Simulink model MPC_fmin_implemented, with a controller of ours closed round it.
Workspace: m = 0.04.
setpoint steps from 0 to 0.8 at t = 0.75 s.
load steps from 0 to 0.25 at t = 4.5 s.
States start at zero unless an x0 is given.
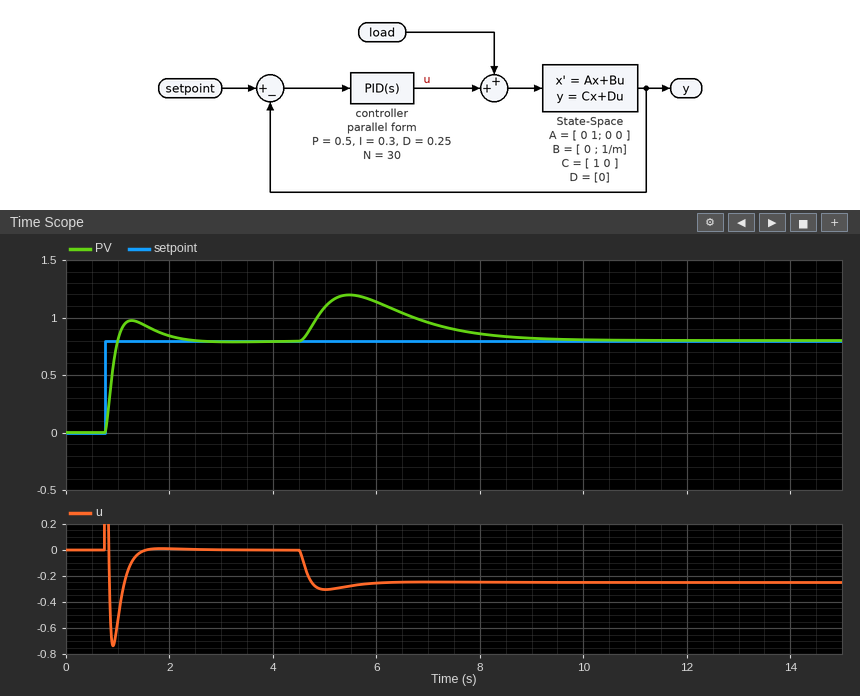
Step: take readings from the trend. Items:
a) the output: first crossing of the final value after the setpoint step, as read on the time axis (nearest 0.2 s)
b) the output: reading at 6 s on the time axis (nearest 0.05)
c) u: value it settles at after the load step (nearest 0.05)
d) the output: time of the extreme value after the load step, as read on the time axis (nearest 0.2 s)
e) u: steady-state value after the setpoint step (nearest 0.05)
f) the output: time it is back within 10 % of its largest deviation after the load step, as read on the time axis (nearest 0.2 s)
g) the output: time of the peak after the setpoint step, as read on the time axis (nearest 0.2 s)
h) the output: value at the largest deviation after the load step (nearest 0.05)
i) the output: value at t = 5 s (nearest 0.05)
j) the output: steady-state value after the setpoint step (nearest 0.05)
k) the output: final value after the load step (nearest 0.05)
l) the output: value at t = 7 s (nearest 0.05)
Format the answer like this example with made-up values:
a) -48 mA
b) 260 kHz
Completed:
a) 1.0 s
b) 1.15
c) -0.25
d) 5.4 s
e) 0.00
f) 8.4 s
g) 1.2 s
h) 1.20
i) 1.10
j) 0.80
k) 0.80
l) 0.95
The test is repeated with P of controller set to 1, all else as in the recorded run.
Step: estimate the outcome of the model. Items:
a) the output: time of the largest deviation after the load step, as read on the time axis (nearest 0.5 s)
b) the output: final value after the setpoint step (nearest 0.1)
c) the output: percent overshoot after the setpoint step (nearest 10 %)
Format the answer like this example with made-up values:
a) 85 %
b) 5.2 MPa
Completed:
a) 5.0 s
b) 0.8
c) 30 %
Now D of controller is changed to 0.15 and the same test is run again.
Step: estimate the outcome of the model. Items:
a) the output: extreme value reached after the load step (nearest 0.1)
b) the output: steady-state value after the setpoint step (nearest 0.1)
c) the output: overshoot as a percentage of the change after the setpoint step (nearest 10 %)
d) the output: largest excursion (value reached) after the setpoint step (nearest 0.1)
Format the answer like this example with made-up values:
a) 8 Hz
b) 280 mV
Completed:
a) 1.3
b) 0.8
c) 40 %
d) 1.1
